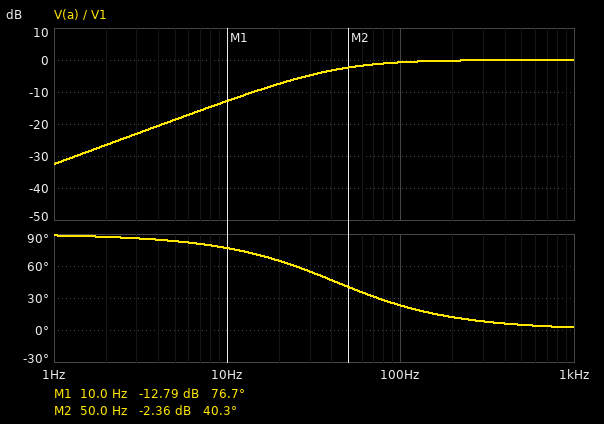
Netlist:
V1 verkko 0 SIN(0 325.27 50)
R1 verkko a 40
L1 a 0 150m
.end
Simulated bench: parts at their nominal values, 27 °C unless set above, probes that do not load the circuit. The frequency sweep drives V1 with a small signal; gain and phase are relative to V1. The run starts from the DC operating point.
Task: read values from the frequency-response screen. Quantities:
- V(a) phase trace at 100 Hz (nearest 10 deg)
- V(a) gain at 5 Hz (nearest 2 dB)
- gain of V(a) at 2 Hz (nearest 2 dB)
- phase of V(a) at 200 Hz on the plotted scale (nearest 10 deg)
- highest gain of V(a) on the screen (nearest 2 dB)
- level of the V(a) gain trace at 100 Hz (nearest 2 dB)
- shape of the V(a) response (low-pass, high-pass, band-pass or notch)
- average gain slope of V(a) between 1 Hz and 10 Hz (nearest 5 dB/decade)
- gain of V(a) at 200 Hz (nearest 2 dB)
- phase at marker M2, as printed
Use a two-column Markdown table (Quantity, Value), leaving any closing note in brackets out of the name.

| Quantity | Value |
|---|---|
| V(a) phase trace at 100 Hz | 20 deg |
| V(a) gain at 5 Hz | -18 dB |
| gain of V(a) at 2 Hz | -26 dB |
| phase of V(a) at 200 Hz on the plotted scale | 10 deg |
| highest gain of V(a) on the screen | 0 dB |
| level of the V(a) gain trace at 100 Hz | 0 dB |
| shape of the V(a) response | high-pass |
| average gain slope of V(a) between 1 Hz and 10 Hz | 20 dB/decade |
| gain of V(a) at 200 Hz | 0 dB |
| phase at marker M2, as printed | 40.3 deg |
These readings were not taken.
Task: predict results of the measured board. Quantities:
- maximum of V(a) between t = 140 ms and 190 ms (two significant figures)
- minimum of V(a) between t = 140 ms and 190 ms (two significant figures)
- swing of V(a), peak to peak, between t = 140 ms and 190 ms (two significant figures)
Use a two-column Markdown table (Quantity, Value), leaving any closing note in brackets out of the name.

| Quantity | Value |
|---|---|
| maximum of V(a) between t = 140 ms and 190 ms | 250 V |
| minimum of V(a) between t = 140 ms and 190 ms | -250 V |
| swing of V(a), peak to peak, between t = 140 ms and 190 ms | 500 V |
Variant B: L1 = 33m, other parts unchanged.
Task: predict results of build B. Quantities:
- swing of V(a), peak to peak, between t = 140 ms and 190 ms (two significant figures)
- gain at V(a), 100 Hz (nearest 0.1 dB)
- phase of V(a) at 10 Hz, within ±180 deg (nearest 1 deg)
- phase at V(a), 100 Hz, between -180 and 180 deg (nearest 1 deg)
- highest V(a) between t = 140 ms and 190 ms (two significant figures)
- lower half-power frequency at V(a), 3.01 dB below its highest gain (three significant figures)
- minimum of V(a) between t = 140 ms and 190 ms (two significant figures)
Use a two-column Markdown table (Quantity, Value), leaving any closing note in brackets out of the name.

| Quantity | Value |
|---|---|
| swing of V(a), peak to peak, between t = 140 ms and 190 ms | 160 V |
| gain at V(a), 100 Hz | -6.7 dB |
| phase of V(a) at 10 Hz, within ±180 deg | 87 deg |
| phase at V(a), 100 Hz, between -180 and 180 deg | 63 deg |
| highest V(a) between t = 140 ms and 190 ms | 82 V |
| lower half-power frequency at V(a), 3.01 dB below its highest gain | 193 Hz |
| minimum of V(a) between t = 140 ms and 190 ms | -82 V |
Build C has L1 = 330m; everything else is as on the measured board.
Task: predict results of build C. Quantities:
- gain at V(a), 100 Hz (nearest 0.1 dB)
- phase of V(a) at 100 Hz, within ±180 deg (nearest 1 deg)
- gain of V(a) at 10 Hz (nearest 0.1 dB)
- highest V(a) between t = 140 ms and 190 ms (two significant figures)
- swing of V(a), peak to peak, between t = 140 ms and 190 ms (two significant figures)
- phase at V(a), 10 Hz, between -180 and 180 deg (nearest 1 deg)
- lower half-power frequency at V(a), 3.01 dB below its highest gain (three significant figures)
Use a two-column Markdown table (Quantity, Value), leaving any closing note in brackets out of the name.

| Quantity | Value |
|---|---|
| gain at V(a), 100 Hz | -0.2 dB |
| phase of V(a) at 100 Hz, within ±180 deg | 11 deg |
| gain of V(a) at 10 Hz | -6.7 dB |
| highest V(a) between t = 140 ms and 190 ms | 300 V |
| swing of V(a), peak to peak, between t = 140 ms and 190 ms | 610 V |
| phase at V(a), 10 Hz, between -180 and 180 deg | 63 deg |
| lower half-power frequency at V(a), 3.01 dB below its highest gain | 19.3 Hz |
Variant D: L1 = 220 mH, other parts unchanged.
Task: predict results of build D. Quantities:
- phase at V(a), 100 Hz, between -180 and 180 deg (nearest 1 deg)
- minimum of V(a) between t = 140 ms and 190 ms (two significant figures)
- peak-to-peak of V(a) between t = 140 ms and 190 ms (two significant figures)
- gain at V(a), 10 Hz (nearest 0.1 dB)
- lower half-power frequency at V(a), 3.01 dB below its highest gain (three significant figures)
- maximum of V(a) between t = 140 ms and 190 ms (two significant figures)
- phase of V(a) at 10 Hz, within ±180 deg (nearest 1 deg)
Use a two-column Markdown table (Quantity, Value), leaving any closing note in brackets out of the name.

| Quantity | Value |
|---|---|
| phase at V(a), 100 Hz, between -180 and 180 deg | 16 deg |
| minimum of V(a) between t = 140 ms and 190 ms | -280 V |
| peak-to-peak of V(a) between t = 140 ms and 190 ms | 560 V |
| gain at V(a), 10 Hz | -9.7 dB |
| lower half-power frequency at V(a), 3.01 dB below its highest gain | 28.9 Hz |
| maximum of V(a) between t = 140 ms and 190 ms | 280 V |
| phase of V(a) at 10 Hz, within ±180 deg | 71 deg |
